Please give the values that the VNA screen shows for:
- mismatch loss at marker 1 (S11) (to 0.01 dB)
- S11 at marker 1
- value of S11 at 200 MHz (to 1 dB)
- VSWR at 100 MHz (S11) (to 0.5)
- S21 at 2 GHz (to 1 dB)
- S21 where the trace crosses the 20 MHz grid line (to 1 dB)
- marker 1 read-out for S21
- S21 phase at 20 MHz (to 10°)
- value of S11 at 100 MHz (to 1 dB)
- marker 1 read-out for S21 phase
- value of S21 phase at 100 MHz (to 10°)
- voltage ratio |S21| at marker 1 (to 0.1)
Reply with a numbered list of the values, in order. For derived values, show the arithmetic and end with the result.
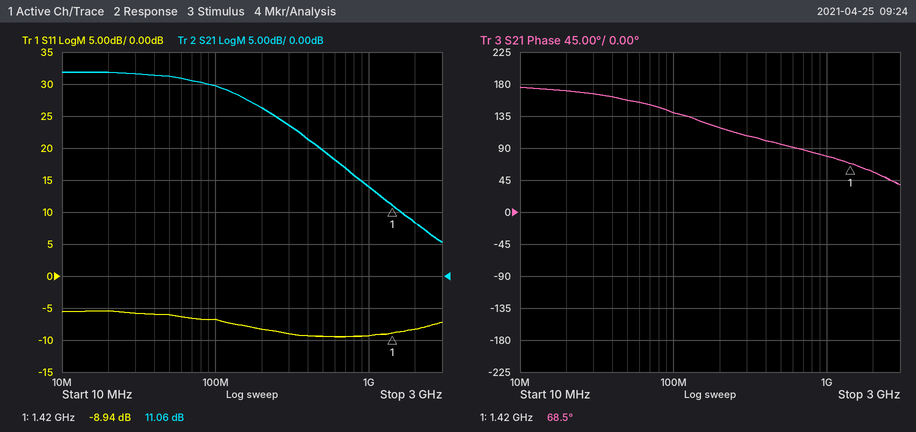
1. −10 log10(1 − 10^(-8.94/10)) ≈ 0.59 dB
2. -8.94 dB
3. -8 dB
4. |Γ| = 10^(-7/20) = 0.4467; VSWR = (1 + 0.4467)/(1 − 0.4467) ≈ 2.61, so 2.5 to the nearest 0.5
5. 8 dB
6. 32 dB
7. 11.06 dB
8. 170°
9. -7 dB
10. 68.5°
11. 140°
12. 10^(11.06/20) ≈ 3.6
